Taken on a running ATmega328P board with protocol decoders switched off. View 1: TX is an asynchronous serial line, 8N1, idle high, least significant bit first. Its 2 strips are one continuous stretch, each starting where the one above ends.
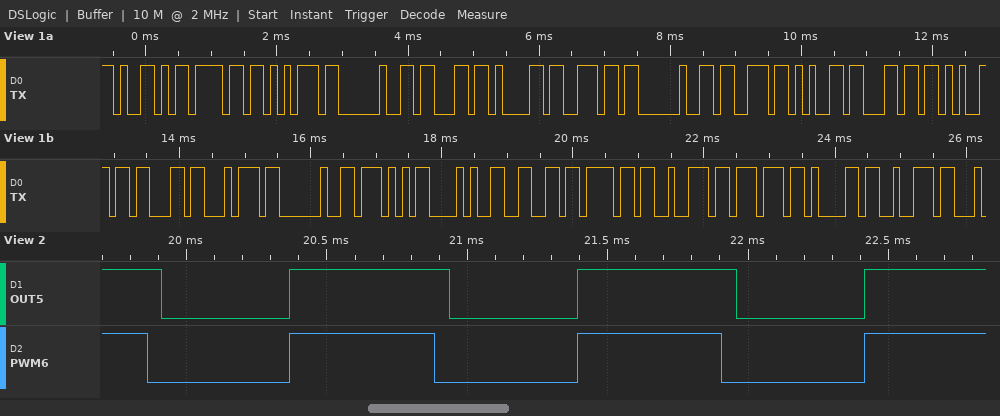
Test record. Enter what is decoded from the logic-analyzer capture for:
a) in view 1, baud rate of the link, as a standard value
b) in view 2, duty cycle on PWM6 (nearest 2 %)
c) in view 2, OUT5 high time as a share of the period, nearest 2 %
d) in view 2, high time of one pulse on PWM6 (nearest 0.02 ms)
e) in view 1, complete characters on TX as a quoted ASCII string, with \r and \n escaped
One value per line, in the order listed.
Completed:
9600 baud
50 %
56 %
0.52 ms
"You can select W(forwar"
